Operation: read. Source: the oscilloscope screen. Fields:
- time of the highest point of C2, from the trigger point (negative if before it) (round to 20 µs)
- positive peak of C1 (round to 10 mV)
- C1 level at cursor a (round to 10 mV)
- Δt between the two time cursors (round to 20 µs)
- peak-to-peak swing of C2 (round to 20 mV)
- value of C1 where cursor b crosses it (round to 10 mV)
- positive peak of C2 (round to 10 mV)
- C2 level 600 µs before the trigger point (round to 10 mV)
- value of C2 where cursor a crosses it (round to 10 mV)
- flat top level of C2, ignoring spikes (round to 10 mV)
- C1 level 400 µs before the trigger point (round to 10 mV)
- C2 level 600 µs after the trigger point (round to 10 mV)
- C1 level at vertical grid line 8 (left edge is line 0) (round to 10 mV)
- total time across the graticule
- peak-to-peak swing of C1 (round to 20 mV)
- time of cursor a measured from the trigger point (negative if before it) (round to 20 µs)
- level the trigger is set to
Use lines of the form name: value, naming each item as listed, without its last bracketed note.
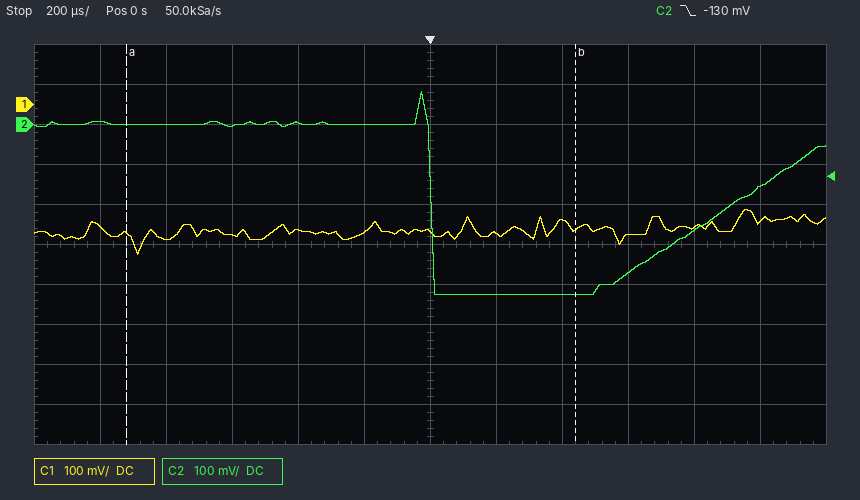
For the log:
time of the highest point of C2, from the trigger point (negative if before it): -20 µs
positive peak of C1: -260 mV
C1 level at cursor a: -320 mV
Δt between the two time cursors: 1.36 ms
peak-to-peak swing of C2: 500 mV
value of C1 where cursor b crosses it: -310 mV
positive peak of C2: 80 mV
C2 level 600 µs before the trigger point: 0 mV
value of C2 where cursor a crosses it: 0 mV
flat top level of C2, ignoring spikes: 0 mV
C1 level 400 µs before the trigger point: -310 mV
C2 level 600 µs after the trigger point: -370 mV
C1 level at vertical grid line 8 (left edge is line 0): -290 mV
total time across the graticule: 2.4 ms
peak-to-peak swing of C1: 120 mV
time of cursor a measured from the trigger point (negative if before it): -920 µs
level the trigger is set to: -130 mV
